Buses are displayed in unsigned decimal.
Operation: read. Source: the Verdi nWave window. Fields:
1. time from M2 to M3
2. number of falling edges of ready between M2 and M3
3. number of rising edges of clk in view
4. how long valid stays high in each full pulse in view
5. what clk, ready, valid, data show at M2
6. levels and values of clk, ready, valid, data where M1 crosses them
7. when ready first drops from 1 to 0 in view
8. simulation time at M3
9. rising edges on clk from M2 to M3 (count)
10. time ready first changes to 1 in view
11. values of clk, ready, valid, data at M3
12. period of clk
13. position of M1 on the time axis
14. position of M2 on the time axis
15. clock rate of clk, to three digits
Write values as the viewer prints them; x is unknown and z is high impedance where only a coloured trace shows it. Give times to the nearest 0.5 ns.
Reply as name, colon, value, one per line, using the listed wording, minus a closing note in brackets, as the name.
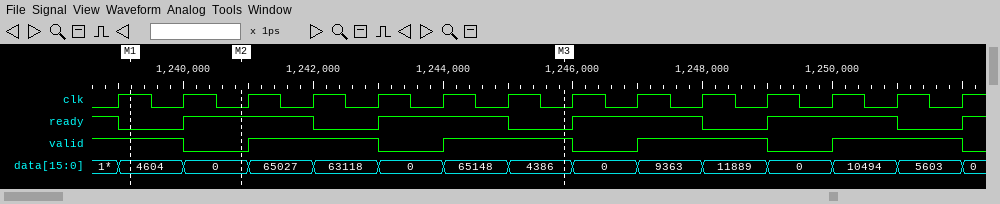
time from M2 to M3: 5 ns
number of falling edges of ready between M2 and M3: 2
number of rising edges of clk in view: 14
how long valid stays high in each full pulse in view: 2 ns, 2 ns, 2 ns, 2 ns
what clk, ready, valid, data show at M2: clk=0, ready=1, valid=0, data=0
levels and values of clk, ready, valid, data where M1 crosses them: clk=1, ready=0, valid=1, data=4604
when ready first drops from 1 to 0 in view: 1239 ns
simulation time at M3: 1246 ns
rising edges on clk from M2 to M3: 5
time ready first changes to 1 in view: 1240 ns
values of clk, ready, valid, data at M3: clk=0, ready=0, valid=1, data=4386
period of clk: 1 ns
position of M1 on the time axis: 1239 ns
position of M2 on the time axis: 1241 ns
clock rate of clk, to three digits: 1.00 GHz
